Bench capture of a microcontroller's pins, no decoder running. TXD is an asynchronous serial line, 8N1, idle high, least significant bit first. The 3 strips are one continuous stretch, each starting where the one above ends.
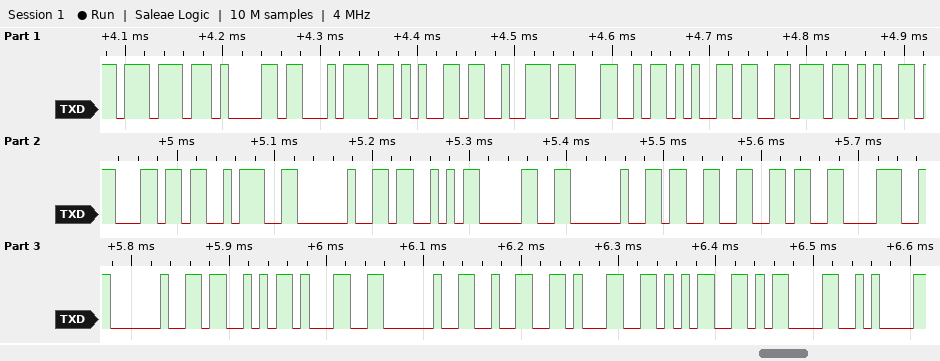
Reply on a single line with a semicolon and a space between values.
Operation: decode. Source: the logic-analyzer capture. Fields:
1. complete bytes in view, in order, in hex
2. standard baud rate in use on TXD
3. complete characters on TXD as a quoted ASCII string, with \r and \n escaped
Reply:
77 61 74 65 72 4C 65 76 65 6C 3A 20 53 30 20 33 36 38 20 53 31 20 32 31 35 0D 0A; 115200 baud; "waterLevel: S0 368 S1 215\r\n"
